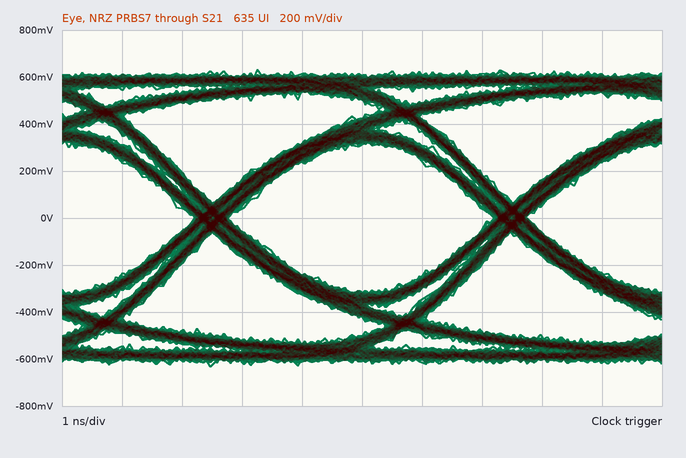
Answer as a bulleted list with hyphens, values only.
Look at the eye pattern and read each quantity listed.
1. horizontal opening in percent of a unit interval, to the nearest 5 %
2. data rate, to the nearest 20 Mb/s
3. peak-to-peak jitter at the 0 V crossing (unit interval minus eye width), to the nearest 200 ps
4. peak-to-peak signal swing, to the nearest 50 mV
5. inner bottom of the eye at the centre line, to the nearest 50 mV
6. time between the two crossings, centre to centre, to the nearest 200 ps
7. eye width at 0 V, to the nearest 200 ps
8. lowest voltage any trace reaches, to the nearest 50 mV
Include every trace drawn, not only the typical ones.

- 90 %
- 200 Mb/s
- 600 ps
- 1.25 V
- -300 mV
- 5.0 ns
- 4.4 ns
- -650 mV
